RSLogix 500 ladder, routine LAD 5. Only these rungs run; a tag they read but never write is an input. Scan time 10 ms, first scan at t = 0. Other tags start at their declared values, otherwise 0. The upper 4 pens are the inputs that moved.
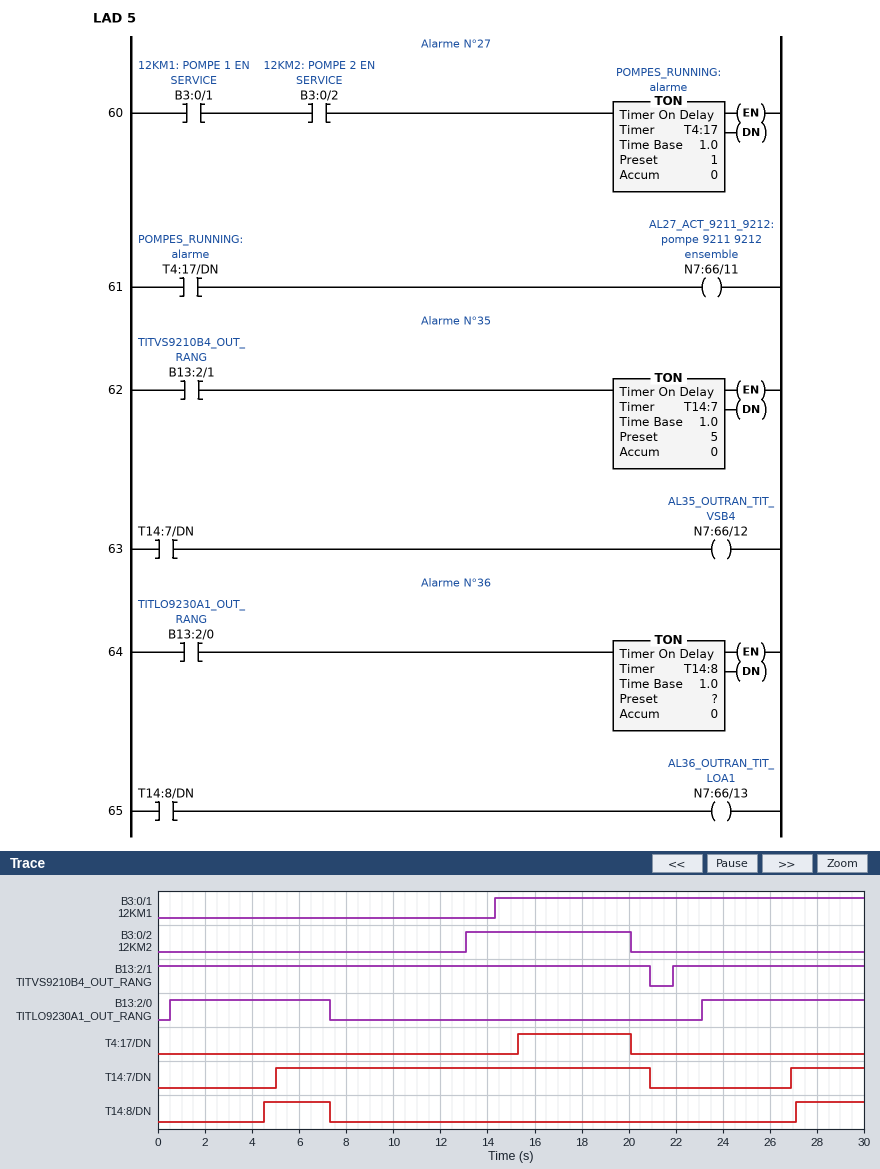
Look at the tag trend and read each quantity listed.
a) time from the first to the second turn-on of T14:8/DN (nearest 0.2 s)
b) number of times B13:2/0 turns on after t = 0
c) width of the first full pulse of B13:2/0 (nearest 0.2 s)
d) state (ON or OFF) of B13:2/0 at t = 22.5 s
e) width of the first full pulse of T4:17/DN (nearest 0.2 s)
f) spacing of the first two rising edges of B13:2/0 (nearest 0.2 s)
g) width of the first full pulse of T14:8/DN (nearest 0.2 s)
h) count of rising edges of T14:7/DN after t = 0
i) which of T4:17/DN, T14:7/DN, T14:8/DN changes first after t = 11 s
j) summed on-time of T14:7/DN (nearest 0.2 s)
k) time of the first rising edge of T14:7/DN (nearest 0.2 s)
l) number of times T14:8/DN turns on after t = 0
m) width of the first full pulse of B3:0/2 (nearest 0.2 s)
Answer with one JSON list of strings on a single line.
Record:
["22.6 s", "2", "6.8 s", "OFF", "4.8 s", "22.6 s", "2.8 s", "2", "T4:17/DN", "19.0 s", "5.0 s", "2", "7.0 s"]
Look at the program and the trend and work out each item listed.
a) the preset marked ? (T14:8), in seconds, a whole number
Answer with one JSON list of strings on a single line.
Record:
["4 s"]
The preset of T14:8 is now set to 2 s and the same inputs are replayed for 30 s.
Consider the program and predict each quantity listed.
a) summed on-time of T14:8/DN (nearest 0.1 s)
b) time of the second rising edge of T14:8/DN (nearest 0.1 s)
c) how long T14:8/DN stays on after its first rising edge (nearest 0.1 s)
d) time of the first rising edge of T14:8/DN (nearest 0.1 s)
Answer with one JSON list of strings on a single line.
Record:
["9.7 s", "25.1 s", "4.8 s", "2.5 s"]
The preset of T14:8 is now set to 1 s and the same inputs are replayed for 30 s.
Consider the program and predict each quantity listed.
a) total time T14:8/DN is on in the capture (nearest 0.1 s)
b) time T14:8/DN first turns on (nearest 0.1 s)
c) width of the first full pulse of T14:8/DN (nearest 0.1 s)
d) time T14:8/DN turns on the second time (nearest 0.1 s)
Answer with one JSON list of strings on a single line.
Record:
["11.7 s", "1.5 s", "5.8 s", "24.1 s"]
